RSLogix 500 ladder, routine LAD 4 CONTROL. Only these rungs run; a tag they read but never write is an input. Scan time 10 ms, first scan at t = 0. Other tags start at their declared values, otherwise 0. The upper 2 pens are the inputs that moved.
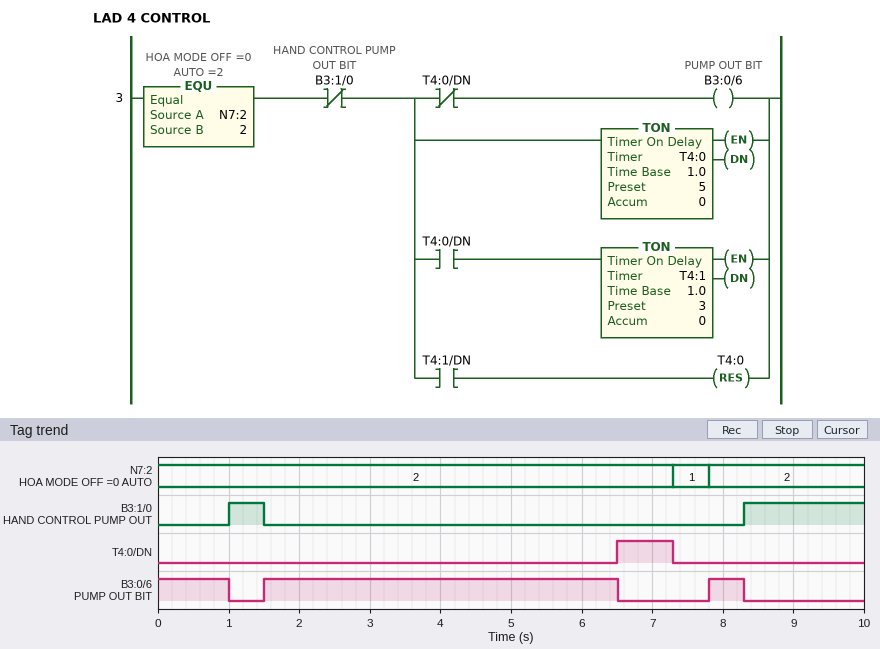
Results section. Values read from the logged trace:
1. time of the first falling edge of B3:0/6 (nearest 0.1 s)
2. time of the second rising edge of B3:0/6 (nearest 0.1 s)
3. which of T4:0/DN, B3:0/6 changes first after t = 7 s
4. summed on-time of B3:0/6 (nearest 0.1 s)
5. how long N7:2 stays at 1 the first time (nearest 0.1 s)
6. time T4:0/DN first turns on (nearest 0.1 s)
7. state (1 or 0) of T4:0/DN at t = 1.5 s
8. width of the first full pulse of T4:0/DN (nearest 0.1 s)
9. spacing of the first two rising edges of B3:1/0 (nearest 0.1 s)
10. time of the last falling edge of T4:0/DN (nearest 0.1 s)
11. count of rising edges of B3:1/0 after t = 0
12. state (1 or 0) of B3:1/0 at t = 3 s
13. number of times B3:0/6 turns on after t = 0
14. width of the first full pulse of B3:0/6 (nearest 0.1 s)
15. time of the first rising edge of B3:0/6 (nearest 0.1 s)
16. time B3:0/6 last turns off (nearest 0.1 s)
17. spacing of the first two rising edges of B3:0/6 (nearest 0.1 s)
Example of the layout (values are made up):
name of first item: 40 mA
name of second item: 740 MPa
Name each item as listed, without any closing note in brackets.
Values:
time of the first falling edge of B3:0/6: 1.0 s
time of the second rising edge of B3:0/6: 7.8 s
which of T4:0/DN, B3:0/6 changes first after t = 7 s: T4:0/DN
summed on-time of B3:0/6: 6.5 s
how long N7:2 stays at 1 the first time: 0.5 s
time T4:0/DN first turns on: 6.5 s
state (1 or 0) of T4:0/DN at t = 1.5 s: 0
width of the first full pulse of T4:0/DN: 0.8 s
spacing of the first two rising edges of B3:1/0: 7.3 s
time of the last falling edge of T4:0/DN: 7.3 s
count of rising edges of B3:1/0 after t = 0: 2
state (1 or 0) of B3:1/0 at t = 3 s: 0
number of times B3:0/6 turns on after t = 0: 2
width of the first full pulse of B3:0/6: 5.0 s
time of the first rising edge of B3:0/6: 1.5 s
time B3:0/6 last turns off: 8.3 s
spacing of the first two rising edges of B3:0/6: 6.3 s
